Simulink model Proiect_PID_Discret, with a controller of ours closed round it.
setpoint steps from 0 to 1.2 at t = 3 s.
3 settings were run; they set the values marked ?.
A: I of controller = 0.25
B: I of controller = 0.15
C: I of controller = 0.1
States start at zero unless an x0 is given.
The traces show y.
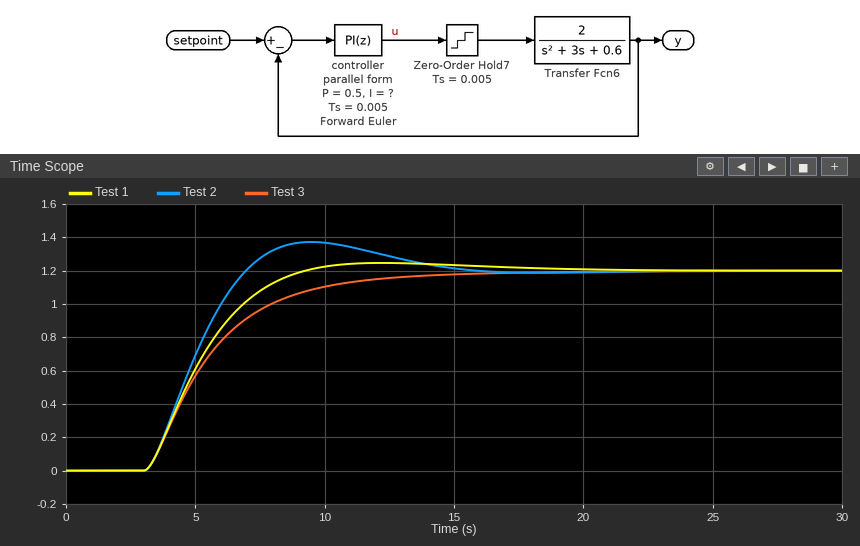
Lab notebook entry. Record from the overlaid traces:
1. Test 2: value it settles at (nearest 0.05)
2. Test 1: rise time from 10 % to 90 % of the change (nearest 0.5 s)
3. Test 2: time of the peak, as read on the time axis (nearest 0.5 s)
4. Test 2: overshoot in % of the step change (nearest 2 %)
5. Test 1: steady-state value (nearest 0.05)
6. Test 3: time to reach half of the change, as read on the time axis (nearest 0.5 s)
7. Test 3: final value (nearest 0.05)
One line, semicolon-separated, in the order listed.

1.20; 4.0 s; 9.5 s; 14 %; 1.20; 5.0 s; 1.20
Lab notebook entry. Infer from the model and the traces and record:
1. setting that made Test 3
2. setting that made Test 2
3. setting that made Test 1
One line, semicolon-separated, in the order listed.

C; A; B
